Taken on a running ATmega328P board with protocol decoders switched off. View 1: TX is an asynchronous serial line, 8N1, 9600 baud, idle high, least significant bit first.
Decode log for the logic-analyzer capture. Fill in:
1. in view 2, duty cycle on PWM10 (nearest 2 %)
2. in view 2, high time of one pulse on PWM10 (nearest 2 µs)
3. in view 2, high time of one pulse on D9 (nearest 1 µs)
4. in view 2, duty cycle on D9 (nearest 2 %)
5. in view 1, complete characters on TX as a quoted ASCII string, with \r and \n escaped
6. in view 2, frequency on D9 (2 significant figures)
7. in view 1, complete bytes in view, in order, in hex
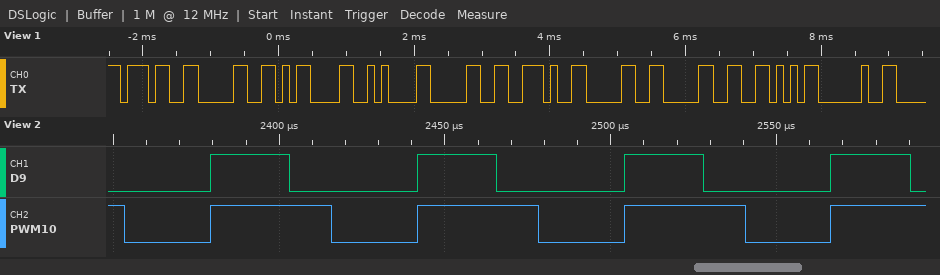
58 %
36 µs
24 µs
38 %
"70\r\n0.00V "
16 kHz
37 30 0D 0A 30 2E 30 30 56 20
